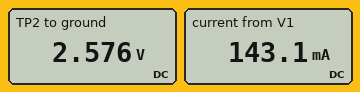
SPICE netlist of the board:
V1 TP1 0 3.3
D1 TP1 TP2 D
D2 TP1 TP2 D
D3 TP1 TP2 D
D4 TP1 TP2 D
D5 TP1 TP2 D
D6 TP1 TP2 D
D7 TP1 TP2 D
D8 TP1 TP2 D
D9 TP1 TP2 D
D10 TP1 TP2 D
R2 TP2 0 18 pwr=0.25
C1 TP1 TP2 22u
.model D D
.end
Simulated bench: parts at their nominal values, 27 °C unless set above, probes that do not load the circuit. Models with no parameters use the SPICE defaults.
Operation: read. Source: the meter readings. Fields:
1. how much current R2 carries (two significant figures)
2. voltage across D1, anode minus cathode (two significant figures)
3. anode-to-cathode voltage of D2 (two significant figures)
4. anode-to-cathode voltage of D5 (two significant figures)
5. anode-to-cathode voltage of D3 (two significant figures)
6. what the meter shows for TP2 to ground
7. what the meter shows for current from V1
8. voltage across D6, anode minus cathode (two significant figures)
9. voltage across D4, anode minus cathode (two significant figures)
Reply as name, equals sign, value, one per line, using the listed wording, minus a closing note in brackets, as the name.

how much current R2 carries = 140 mA
voltage across D1, anode minus cathode = 720 mV
anode-to-cathode voltage of D2 = 720 mV
anode-to-cathode voltage of D5 = 720 mV
anode-to-cathode voltage of D3 = 720 mV
what the meter shows for TP2 to ground = 2.576 V
what the meter shows for current from V1 = 143.1 mA
voltage across D6, anode minus cathode = 720 mV
voltage across D4, anode minus cathode = 720 mV
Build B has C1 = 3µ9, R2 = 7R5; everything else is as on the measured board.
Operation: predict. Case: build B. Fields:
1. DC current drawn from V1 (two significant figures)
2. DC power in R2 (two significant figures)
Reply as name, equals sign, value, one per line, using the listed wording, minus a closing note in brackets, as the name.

DC current drawn from V1 = 340 mA
DC power in R2 = 870 mW
